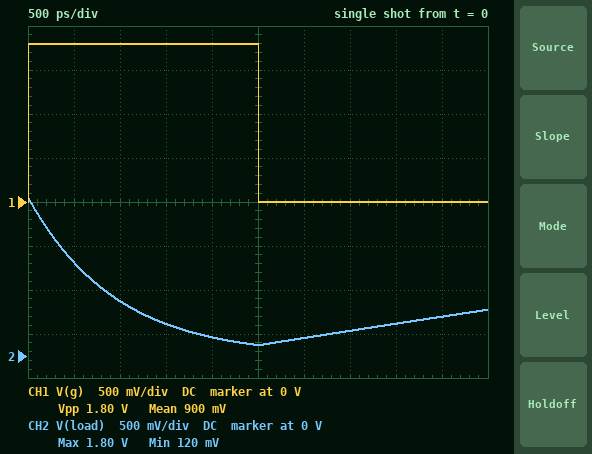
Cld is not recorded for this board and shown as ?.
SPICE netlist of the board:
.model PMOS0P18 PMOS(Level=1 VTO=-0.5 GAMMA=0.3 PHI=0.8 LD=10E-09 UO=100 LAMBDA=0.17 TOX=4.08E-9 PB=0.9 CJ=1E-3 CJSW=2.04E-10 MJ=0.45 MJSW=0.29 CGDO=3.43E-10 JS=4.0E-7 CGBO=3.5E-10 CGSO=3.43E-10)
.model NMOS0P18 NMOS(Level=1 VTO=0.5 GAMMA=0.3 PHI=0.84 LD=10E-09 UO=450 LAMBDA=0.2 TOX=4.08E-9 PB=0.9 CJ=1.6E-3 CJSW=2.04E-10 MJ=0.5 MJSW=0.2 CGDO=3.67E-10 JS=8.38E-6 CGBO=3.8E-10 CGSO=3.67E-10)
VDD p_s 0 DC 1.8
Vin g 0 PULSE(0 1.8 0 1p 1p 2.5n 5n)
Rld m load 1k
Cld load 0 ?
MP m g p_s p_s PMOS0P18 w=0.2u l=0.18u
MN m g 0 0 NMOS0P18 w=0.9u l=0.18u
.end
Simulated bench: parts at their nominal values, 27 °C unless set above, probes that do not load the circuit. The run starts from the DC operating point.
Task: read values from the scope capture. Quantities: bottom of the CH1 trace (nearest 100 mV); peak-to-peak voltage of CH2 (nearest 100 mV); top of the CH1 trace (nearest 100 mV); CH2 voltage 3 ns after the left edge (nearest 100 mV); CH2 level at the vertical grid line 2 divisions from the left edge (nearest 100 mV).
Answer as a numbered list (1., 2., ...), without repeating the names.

1. 0 V
2. 1.7 V
3. 1.8 V
4. 200 mV
5. 600 mV
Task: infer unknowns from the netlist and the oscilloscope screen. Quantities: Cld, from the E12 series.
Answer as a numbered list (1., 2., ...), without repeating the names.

1. 680 fF
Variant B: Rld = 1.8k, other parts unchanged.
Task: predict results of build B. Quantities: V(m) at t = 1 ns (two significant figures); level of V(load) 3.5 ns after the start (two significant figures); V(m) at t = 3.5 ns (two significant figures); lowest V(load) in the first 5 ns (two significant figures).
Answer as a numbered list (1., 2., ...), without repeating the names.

1. 160 mV
2. 490 mV
3. 670 mV
4. 330 mV
